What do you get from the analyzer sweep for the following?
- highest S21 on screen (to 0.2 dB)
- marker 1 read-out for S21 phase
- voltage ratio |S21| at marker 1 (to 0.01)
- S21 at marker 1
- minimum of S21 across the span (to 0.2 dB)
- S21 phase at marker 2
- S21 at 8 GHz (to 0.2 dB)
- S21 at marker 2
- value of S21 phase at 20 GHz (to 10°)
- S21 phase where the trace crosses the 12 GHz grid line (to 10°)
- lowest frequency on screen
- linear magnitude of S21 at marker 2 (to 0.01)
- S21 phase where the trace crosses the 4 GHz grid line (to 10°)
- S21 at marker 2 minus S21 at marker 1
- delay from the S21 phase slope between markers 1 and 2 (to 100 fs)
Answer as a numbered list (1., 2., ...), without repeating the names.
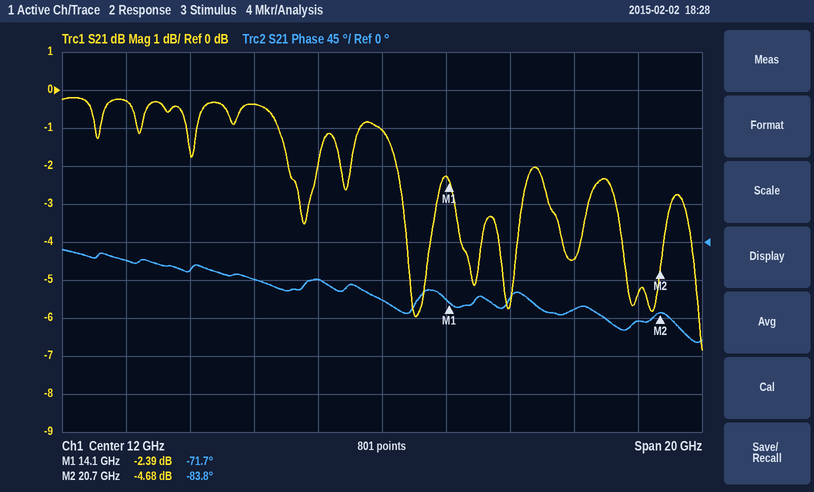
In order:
1. -0.2 dB
2. -71.7°
3. 0.76
4. -2.39 dB
5. -6.8 dB
6. -83.8°
7. -0.4 dB
8. -4.68 dB
9. -90°
10. -70°
11. 2 GHz
12. 0.58
13. -20°
14. -2.29 dB
15. 5.1 ps
